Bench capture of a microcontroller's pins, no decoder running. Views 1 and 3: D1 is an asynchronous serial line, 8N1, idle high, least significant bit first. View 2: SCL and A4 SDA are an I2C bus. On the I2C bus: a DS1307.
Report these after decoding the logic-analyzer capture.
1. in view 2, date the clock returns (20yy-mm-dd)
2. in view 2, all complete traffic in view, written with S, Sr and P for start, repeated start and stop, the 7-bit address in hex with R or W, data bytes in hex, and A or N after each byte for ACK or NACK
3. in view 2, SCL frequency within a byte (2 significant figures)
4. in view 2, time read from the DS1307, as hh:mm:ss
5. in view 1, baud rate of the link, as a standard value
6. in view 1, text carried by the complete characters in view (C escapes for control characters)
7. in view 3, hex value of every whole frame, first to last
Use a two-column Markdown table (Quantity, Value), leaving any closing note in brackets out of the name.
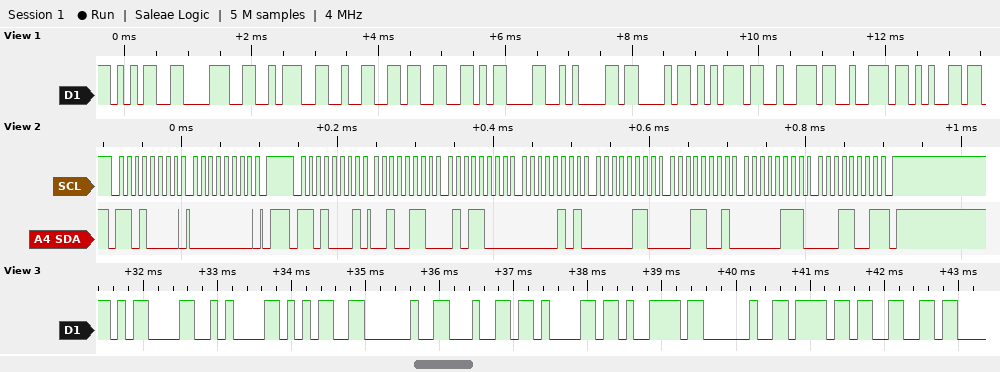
| Quantity | Value |
|---|---|
| in view 2, date the clock returns | 2019-07-19 |
| in view 2, all complete traffic in view, written with S, Sr and P for start, repeated start and stop, the 7-bit address in hex with R or W, data bytes in hex, and A or N after each byte for ACK or NACK | S 68W A 00 A P S 68R A 26 A 58 A 05 A 06 A 19 A 07 A 19 N P |
| in view 2, SCL frequency within a byte | 100 kHz |
| in view 2, time read from the DS1307, as hh:mm:ss | 05:58:26 |
| in view 1, baud rate of the link, as a standard value | 9600 baud |
| in view 1, text carried by the complete characters in view | "58:23\r\nCurre" |
| in view 3, hex value of every whole frame, first to last | 0x0D 0x0A 0x35 0x20 0x64 0x61 0x79 0x20 0x6F 0x66 |
